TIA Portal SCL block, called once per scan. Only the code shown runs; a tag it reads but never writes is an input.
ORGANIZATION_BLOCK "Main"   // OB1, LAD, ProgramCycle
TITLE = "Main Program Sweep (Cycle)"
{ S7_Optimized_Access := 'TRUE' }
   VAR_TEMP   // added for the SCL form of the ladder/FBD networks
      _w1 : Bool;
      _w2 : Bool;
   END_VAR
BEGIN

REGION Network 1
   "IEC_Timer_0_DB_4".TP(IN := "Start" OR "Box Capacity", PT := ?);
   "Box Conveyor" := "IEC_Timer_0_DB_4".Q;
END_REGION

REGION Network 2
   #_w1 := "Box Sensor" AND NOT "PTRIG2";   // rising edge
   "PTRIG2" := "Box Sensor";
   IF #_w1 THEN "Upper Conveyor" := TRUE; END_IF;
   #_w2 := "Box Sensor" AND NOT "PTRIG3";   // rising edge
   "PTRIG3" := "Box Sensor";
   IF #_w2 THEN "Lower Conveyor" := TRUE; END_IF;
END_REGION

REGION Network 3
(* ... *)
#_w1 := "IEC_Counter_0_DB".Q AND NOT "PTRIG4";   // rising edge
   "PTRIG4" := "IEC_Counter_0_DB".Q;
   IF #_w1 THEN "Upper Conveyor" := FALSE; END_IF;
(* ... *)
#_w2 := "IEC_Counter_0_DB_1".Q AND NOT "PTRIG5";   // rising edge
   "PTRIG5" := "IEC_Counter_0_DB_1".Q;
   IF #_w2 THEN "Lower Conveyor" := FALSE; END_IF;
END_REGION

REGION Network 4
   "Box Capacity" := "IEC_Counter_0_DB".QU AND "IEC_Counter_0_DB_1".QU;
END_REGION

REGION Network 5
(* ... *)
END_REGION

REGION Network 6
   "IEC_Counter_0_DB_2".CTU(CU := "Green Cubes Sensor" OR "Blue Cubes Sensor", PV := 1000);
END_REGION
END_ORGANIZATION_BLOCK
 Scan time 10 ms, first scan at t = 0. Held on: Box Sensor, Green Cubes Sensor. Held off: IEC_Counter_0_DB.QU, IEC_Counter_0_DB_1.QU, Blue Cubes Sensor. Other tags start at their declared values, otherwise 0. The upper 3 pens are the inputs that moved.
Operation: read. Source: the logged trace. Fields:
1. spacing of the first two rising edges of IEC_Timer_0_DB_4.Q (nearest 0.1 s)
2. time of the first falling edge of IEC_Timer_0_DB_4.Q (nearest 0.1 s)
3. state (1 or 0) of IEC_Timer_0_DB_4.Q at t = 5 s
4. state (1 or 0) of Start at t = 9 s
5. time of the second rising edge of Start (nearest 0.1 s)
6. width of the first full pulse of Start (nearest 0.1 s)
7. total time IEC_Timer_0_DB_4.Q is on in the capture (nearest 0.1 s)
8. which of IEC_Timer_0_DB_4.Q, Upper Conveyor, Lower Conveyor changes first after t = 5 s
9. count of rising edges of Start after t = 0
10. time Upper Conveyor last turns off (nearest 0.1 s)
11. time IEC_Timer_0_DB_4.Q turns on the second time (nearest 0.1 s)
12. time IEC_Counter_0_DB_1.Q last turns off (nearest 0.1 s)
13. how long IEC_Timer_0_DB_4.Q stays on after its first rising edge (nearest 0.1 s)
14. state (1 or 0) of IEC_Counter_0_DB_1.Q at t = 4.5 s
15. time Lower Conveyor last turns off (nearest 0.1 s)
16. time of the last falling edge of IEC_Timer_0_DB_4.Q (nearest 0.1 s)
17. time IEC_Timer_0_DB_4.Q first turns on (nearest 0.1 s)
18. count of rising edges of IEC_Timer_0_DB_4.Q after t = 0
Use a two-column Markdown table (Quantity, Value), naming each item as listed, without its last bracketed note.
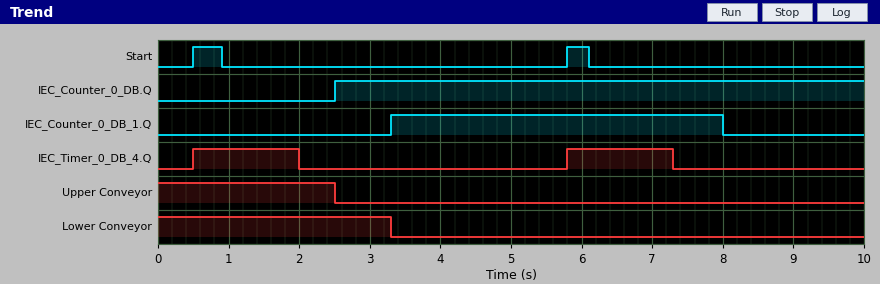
| Quantity | Value |
|---|---|
| spacing of the first two rising edges of IEC_Timer_0_DB_4.Q | 5.3 s |
| time of the first falling edge of IEC_Timer_0_DB_4.Q | 2.0 s |
| state (1 or 0) of IEC_Timer_0_DB_4.Q at t = 5 s | 0 |
| state (1 or 0) of Start at t = 9 s | 0 |
| time of the second rising edge of Start | 5.8 s |
| width of the first full pulse of Start | 0.4 s |
| total time IEC_Timer_0_DB_4.Q is on in the capture | 3.0 s |
| which of IEC_Timer_0_DB_4.Q, Upper Conveyor, Lower Conveyor changes first after t = 5 s | IEC_Timer_0_DB_4.Q |
| count of rising edges of Start after t = 0 | 2 |
| time Upper Conveyor last turns off | 2.5 s |
| time IEC_Timer_0_DB_4.Q turns on the second time | 5.8 s |
| time IEC_Counter_0_DB_1.Q last turns off | 8.0 s |
| how long IEC_Timer_0_DB_4.Q stays on after its first rising edge | 1.5 s |
| state (1 or 0) of IEC_Counter_0_DB_1.Q at t = 4.5 s | 1 |
| time Lower Conveyor last turns off | 3.3 s |
| time of the last falling edge of IEC_Timer_0_DB_4.Q | 7.3 s |
| time IEC_Timer_0_DB_4.Q first turns on | 0.5 s |
| count of rising edges of IEC_Timer_0_DB_4.Q after t = 0 | 2 |
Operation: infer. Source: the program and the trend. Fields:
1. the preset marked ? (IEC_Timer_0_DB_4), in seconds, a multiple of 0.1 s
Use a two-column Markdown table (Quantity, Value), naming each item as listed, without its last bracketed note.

| Quantity | Value |
|---|---|
| the preset marked ? (IEC_Timer_0_DB_4), in seconds, a multiple of 0.1 s | 1.5 s |
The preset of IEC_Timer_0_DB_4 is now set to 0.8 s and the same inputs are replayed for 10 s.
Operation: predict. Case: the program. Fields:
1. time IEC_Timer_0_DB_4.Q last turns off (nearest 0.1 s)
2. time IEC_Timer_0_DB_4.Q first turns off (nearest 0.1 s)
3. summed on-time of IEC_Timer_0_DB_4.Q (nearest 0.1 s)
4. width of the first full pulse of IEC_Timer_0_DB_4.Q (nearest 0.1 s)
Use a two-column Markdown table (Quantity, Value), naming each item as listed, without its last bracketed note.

| Quantity | Value |
|---|---|
| time IEC_Timer_0_DB_4.Q last turns off | 6.6 s |
| time IEC_Timer_0_DB_4.Q first turns off | 1.3 s |
| summed on-time of IEC_Timer_0_DB_4.Q | 1.6 s |
| width of the first full pulse of IEC_Timer_0_DB_4.Q | 0.8 s |
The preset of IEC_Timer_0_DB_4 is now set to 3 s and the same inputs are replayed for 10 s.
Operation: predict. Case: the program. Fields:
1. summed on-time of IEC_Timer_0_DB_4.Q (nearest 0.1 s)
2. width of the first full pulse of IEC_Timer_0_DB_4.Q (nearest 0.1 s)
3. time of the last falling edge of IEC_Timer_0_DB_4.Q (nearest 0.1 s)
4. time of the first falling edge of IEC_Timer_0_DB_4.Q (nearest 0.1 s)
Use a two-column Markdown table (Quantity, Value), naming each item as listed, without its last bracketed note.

| Quantity | Value |
|---|---|
| summed on-time of IEC_Timer_0_DB_4.Q | 6.0 s |
| width of the first full pulse of IEC_Timer_0_DB_4.Q | 3.0 s |
| time of the last falling edge of IEC_Timer_0_DB_4.Q | 8.8 s |
| time of the first falling edge of IEC_Timer_0_DB_4.Q | 3.5 s |
